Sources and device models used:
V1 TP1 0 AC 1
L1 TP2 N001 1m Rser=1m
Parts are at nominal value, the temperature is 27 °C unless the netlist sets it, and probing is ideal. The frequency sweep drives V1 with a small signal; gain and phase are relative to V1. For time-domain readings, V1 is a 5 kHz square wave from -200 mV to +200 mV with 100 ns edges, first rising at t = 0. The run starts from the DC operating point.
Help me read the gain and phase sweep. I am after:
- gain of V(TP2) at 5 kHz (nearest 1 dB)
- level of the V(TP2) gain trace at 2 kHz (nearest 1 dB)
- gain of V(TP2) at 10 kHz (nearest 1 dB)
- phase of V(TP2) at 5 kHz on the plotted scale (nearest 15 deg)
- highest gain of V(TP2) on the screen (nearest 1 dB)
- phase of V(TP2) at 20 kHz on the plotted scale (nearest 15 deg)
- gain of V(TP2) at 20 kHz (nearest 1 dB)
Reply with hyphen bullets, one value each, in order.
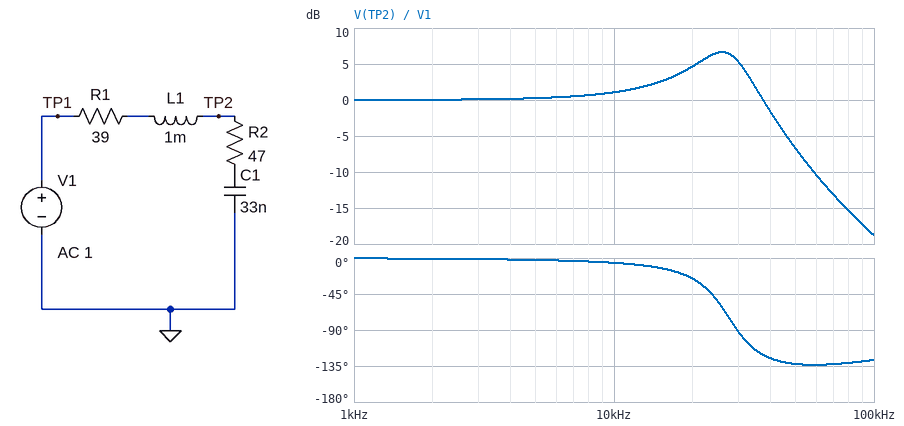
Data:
- 0 dB
- 0 dB
- 1 dB
- 0 deg
- 7 dB
- -30 deg
- 5 dB
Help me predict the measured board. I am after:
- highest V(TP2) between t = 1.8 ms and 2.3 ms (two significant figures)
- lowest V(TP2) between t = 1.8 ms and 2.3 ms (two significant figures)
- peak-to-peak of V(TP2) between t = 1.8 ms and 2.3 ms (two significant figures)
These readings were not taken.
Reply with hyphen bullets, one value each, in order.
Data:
- 390 mV
- -390 mV
- 780 mV
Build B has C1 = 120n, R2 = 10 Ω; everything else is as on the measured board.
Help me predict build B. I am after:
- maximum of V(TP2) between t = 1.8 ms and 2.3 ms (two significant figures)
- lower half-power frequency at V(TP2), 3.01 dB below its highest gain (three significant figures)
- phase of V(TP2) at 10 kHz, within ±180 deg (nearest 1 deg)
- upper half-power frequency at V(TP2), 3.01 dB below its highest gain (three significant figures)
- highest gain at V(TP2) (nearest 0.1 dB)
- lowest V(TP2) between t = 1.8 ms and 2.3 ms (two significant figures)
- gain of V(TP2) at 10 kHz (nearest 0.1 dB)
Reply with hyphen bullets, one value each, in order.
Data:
- 380 mV
- 8.50 kHz
- -31 deg
- 17.0 kHz
- 5.8 dB
- -380 mV
- 3.9 dB
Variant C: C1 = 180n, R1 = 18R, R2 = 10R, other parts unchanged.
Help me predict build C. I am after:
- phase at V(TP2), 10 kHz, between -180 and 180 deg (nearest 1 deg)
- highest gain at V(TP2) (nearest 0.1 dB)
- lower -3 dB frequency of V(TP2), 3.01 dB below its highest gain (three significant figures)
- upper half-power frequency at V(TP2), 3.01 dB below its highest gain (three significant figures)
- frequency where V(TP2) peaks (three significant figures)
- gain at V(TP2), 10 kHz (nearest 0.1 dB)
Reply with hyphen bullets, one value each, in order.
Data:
- -41 deg
- 8.7 dB
- 8.90 kHz
- 13.5 kHz
- 11.4 kHz
- 7.4 dB
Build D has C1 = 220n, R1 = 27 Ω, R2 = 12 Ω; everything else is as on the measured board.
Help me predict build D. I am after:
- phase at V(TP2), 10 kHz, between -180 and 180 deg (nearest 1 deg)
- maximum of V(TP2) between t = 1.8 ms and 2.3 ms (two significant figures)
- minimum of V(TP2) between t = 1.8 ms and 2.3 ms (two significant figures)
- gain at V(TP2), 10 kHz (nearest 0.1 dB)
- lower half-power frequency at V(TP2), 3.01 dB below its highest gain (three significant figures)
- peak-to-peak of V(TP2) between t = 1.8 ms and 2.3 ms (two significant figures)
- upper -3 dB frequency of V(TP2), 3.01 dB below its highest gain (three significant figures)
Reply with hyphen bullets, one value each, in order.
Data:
- -67 deg
- 340 mV
- -340 mV
- 5.2 dB
- 5.76 kHz
- 670 mV
- 12.7 kHz
